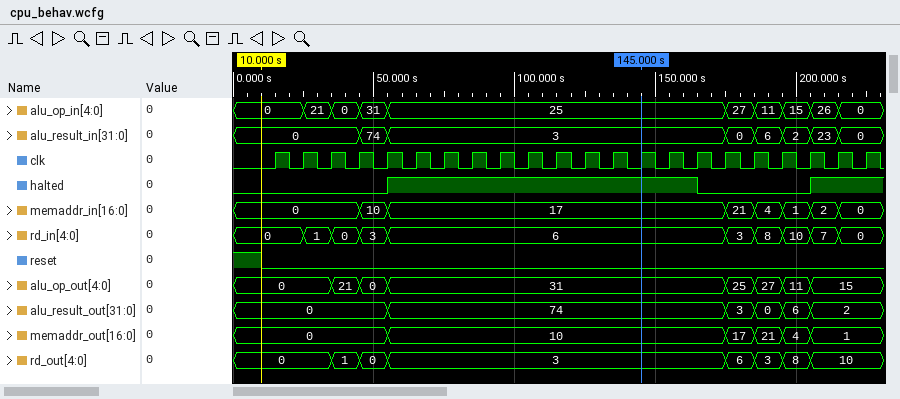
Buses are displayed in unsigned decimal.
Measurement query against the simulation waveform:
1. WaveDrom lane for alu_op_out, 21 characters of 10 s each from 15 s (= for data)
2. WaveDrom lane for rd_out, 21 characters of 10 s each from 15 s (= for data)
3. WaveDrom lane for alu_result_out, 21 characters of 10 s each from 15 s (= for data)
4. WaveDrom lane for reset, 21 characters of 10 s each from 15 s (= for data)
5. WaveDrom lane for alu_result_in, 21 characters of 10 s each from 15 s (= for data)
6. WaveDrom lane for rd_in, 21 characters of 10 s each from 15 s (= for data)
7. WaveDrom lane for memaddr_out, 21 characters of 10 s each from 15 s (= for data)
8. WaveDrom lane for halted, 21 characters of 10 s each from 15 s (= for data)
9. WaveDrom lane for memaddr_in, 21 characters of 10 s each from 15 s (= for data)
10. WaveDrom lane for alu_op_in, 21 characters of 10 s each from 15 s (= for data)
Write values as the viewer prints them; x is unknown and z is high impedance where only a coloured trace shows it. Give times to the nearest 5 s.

{name: 'alu_op_out', wave: '=.===...........====.', data: '0 21 0 31 25 27 11 15'}
{name: 'rd_out', wave: '=.===...........====.', data: '0 1 0 3 6 3 8 10'}
{name: 'alu_result_out', wave: '=...=...........====.', data: '0 74 3 0 6 2'}
{name: 'reset', wave: '0....................'}
{name: 'alu_result_in', wave: '=..==...........=====', data: '0 74 3 0 6 2 23 0'}
{name: 'rd_in', wave: '=====...........=====', data: '0 1 0 3 6 3 8 10 7 0'}
{name: 'memaddr_out', wave: '=...=...........====.', data: '0 10 17 21 4 1'}
{name: 'halted', wave: '0...1..........0...1.'}
{name: 'memaddr_in', wave: '=..==...........=====', data: '0 10 17 21 4 1 2 0'}
{name: 'alu_op_in', wave: '=====...........=====', data: '0 21 0 31 25 27 11 15 26 0'}
